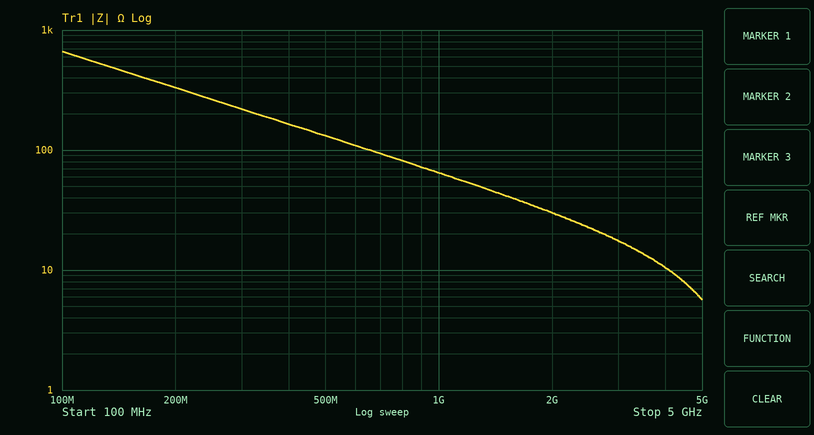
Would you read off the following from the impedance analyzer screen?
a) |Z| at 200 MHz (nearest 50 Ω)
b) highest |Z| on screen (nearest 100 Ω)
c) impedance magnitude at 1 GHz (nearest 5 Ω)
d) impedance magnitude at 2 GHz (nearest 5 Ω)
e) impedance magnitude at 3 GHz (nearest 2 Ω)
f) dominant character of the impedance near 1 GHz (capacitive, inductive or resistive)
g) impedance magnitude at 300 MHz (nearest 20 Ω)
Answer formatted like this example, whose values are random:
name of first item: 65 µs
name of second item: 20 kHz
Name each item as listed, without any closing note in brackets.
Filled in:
|Z| at 200 MHz: 350 Ω
highest |Z| on screen: 700 Ω
impedance magnitude at 1 GHz: 65 Ω
impedance magnitude at 2 GHz: 30 Ω
impedance magnitude at 3 GHz: 18 Ω
dominant character of the impedance near 1 GHz: capacitive
impedance magnitude at 300 MHz: 220 Ω
